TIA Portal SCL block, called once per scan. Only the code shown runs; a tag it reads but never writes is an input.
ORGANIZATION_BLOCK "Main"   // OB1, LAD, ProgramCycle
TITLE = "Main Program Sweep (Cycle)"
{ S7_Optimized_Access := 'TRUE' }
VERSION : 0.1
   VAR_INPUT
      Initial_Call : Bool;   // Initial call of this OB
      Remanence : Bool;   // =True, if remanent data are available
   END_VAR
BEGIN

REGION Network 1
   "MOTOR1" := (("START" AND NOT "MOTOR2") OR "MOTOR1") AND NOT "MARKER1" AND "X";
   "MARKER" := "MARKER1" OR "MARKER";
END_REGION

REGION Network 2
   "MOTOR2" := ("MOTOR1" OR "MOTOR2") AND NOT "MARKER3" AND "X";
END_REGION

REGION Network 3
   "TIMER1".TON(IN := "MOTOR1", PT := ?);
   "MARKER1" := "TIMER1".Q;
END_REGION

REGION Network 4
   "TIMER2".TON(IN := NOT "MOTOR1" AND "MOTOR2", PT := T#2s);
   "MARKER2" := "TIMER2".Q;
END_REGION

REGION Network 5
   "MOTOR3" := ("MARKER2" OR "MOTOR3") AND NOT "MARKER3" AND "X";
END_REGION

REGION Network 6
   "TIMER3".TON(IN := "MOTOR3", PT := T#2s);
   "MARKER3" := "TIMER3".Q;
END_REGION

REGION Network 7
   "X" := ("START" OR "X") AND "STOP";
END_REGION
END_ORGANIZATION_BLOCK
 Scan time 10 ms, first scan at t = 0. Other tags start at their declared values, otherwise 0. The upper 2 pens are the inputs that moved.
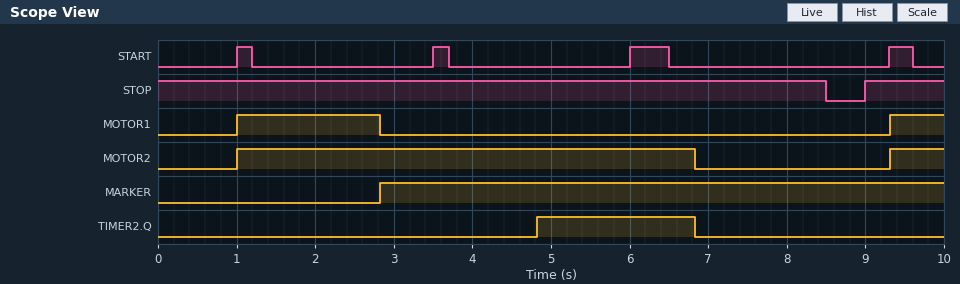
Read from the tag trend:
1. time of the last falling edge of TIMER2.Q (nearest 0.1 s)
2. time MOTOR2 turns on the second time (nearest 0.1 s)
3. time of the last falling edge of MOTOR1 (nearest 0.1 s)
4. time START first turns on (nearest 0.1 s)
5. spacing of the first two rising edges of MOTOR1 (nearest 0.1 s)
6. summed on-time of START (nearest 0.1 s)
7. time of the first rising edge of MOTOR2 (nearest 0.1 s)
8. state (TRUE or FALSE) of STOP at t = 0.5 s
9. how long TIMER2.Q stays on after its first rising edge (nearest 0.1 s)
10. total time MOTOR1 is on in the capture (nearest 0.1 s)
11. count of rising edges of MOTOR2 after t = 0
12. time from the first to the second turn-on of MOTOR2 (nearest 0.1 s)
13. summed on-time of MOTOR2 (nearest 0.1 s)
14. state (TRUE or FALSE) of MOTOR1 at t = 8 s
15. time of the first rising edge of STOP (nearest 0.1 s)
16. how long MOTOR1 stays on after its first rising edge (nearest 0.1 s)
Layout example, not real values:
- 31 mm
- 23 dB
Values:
- 6.8 s
- 9.3 s
- 2.8 s
- 1.0 s
- 8.3 s
- 1.2 s
- 1.0 s
- TRUE
- 2.0 s
- 2.5 s
- 2
- 8.3 s
- 6.5 s
- FALSE
- 9.0 s
- 1.8 s
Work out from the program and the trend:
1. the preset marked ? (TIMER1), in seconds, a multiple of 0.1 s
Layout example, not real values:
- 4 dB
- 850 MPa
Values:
- 1.8 s
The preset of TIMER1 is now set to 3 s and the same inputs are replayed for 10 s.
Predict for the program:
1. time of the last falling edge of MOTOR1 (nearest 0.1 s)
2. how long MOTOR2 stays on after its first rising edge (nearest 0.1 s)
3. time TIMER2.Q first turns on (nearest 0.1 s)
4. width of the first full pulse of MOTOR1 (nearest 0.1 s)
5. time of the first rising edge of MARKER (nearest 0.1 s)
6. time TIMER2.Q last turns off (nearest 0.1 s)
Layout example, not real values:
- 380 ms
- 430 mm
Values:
- 4.0 s
- 7.0 s
- 6.0 s
- 3.0 s
- 4.0 s
- 8.0 s
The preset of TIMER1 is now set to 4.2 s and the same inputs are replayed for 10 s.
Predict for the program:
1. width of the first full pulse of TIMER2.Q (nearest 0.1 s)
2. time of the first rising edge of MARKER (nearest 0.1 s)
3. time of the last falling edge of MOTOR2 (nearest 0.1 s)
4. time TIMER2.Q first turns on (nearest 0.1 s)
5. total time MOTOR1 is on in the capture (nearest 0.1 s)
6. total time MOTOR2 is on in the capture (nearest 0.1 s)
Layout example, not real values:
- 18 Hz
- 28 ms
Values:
- 1.3 s
- 5.2 s
- 8.5 s
- 7.2 s
- 4.9 s
- 8.2 s
